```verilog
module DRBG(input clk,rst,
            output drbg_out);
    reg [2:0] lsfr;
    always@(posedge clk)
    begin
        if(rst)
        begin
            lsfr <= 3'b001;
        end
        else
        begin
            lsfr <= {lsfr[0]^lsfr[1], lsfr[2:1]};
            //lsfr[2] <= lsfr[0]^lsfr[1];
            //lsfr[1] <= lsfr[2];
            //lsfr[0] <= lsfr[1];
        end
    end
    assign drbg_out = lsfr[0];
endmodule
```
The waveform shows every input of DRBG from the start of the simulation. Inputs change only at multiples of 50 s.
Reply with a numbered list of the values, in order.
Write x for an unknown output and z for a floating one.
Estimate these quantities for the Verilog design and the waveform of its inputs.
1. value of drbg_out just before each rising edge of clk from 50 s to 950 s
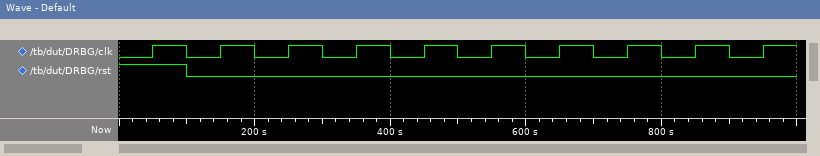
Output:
1. x 1 0 0 1 0 1 1 1 0
